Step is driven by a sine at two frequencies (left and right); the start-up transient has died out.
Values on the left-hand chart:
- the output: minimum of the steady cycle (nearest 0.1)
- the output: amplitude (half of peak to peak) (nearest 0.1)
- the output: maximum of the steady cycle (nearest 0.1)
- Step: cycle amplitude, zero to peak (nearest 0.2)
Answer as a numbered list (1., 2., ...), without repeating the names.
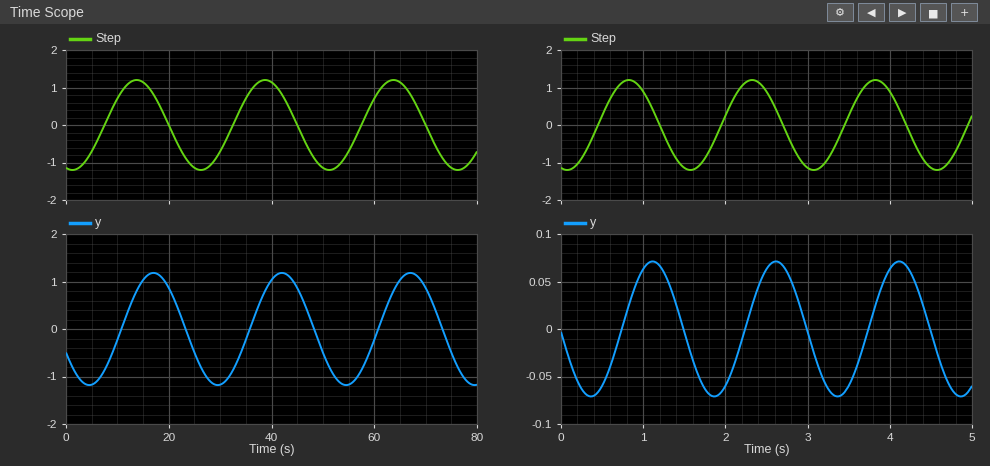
1. -1.2
2. 1.2
3. 1.2
4. 1.2
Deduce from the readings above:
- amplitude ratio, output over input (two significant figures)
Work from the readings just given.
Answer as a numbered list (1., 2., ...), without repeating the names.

1. 1.0
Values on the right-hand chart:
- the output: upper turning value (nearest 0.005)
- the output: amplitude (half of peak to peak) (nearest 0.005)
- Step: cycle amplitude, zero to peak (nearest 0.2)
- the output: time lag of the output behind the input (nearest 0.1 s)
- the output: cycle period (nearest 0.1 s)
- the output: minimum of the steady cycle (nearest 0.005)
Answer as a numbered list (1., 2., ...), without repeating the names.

1. 0.070
2. 0.070
3. 1.2
4. 0.3 s
5. 1.5 s
6. -0.070
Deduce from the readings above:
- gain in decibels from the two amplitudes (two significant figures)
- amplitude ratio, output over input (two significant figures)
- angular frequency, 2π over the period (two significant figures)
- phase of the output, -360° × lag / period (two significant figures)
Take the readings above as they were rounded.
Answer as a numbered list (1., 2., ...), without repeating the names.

1. -25 dB
2. 0.058
3. 4.2 rad/s
4. -72°
